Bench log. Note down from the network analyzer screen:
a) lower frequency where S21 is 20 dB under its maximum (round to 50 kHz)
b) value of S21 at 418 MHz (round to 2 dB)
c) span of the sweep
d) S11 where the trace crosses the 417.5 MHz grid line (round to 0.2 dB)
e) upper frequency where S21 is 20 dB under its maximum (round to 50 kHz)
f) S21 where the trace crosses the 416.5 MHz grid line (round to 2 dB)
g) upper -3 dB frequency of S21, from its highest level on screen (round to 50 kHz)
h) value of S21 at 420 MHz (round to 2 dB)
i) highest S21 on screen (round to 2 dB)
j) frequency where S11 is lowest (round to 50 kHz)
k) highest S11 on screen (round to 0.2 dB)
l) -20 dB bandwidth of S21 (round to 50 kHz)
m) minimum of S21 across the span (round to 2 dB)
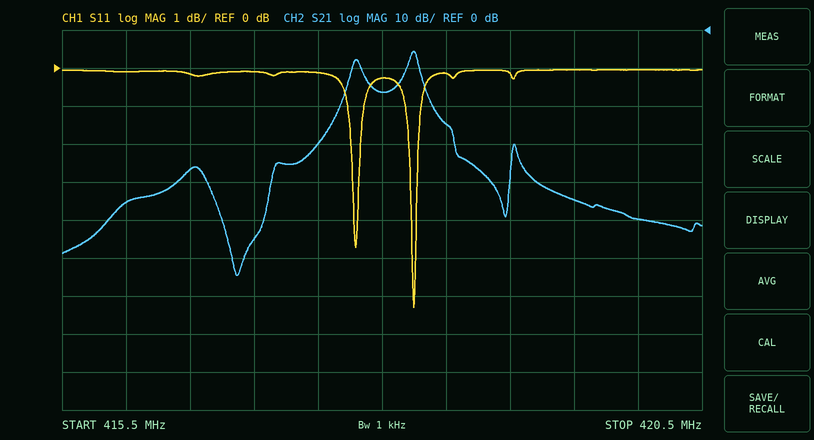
417.60 MHz
-16 dB
5 MHz
-0.2 dB
418.55 MHz
-36 dB
418.30 MHz
-50 dB
-6 dB
418.25 MHz
0.0 dB
950 kHz
-64 dB
